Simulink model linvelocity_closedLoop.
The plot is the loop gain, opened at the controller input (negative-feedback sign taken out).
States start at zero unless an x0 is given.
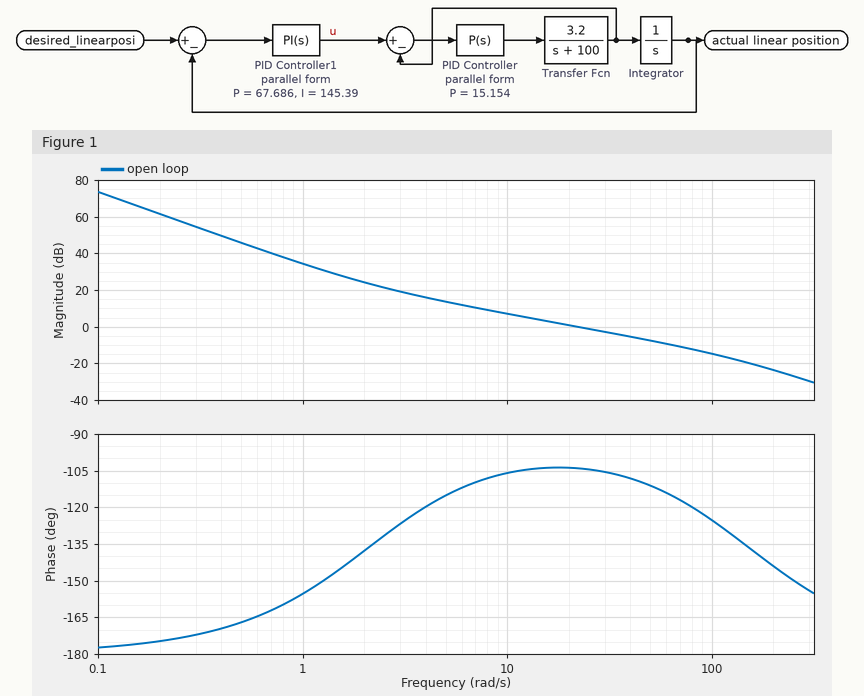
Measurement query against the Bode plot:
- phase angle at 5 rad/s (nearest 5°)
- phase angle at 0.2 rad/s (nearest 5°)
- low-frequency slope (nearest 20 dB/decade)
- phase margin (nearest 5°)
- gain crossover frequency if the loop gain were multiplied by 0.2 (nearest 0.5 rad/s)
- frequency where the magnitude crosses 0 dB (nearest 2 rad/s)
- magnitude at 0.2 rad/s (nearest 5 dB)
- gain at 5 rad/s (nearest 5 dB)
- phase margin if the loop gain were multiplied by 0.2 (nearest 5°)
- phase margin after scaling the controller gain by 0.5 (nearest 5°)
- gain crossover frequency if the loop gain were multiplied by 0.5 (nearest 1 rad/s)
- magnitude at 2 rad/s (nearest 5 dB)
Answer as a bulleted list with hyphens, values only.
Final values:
- -115°
- -175°
- -40 dB/decade
- 75°
- 5.0 rad/s
- 22 rad/s
- 60 dB
- 15 dB
- 65°
- 75°
- 11 rad/s
- 25 dB
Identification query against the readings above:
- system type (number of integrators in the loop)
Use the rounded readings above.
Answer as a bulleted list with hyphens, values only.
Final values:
- 2
